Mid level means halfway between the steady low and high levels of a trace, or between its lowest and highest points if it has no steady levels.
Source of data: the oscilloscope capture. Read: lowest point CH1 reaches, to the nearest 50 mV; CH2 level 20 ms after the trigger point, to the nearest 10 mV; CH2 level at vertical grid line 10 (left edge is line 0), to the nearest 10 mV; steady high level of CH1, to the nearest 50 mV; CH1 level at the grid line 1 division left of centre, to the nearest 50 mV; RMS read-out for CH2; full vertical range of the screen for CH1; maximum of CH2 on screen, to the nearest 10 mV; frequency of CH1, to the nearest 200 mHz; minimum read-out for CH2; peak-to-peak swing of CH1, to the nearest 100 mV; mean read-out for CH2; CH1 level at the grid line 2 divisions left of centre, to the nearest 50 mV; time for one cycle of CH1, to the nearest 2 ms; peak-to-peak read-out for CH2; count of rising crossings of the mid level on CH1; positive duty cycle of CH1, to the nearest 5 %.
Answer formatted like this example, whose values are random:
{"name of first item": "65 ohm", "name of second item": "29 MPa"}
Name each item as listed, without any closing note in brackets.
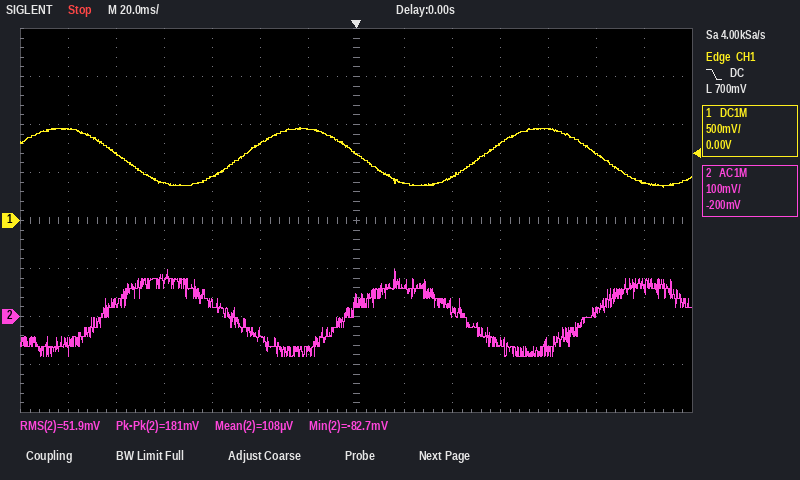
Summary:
{"lowest point CH1 reaches, to the nearest 50 mV": "350 mV", "CH2 level 20 ms after the trigger point, to the nearest 10 mV": "60 mV", "CH2 level at vertical grid line 10 (left edge is line 0), to the nearest 10 mV": "-50 mV", "steady high level of CH1, to the nearest 50 mV": "950 mV", "CH1 level at the grid line 1 division left of centre, to the nearest 50 mV": "950 mV", "RMS read-out for CH2": "51.9 mV", "full vertical range of the screen for CH1": "4 V", "maximum of CH2 on screen, to the nearest 10 mV": "100 mV", "frequency of CH1, to the nearest 200 mHz": "10.0 Hz", "minimum read-out for CH2": "-82.7 mV", "peak-to-peak swing of CH1, to the nearest 100 mV": "600 mV", "mean read-out for CH2": "108 µV", "CH1 level at the grid line 2 divisions left of centre, to the nearest 50 mV": "800 mV", "time for one cycle of CH1, to the nearest 2 ms": "100 ms", "peak-to-peak read-out for CH2": "181 mV", "count of rising crossings of the mid level on CH1": "2", "positive duty cycle of CH1, to the nearest 5 %": "50 %"}
